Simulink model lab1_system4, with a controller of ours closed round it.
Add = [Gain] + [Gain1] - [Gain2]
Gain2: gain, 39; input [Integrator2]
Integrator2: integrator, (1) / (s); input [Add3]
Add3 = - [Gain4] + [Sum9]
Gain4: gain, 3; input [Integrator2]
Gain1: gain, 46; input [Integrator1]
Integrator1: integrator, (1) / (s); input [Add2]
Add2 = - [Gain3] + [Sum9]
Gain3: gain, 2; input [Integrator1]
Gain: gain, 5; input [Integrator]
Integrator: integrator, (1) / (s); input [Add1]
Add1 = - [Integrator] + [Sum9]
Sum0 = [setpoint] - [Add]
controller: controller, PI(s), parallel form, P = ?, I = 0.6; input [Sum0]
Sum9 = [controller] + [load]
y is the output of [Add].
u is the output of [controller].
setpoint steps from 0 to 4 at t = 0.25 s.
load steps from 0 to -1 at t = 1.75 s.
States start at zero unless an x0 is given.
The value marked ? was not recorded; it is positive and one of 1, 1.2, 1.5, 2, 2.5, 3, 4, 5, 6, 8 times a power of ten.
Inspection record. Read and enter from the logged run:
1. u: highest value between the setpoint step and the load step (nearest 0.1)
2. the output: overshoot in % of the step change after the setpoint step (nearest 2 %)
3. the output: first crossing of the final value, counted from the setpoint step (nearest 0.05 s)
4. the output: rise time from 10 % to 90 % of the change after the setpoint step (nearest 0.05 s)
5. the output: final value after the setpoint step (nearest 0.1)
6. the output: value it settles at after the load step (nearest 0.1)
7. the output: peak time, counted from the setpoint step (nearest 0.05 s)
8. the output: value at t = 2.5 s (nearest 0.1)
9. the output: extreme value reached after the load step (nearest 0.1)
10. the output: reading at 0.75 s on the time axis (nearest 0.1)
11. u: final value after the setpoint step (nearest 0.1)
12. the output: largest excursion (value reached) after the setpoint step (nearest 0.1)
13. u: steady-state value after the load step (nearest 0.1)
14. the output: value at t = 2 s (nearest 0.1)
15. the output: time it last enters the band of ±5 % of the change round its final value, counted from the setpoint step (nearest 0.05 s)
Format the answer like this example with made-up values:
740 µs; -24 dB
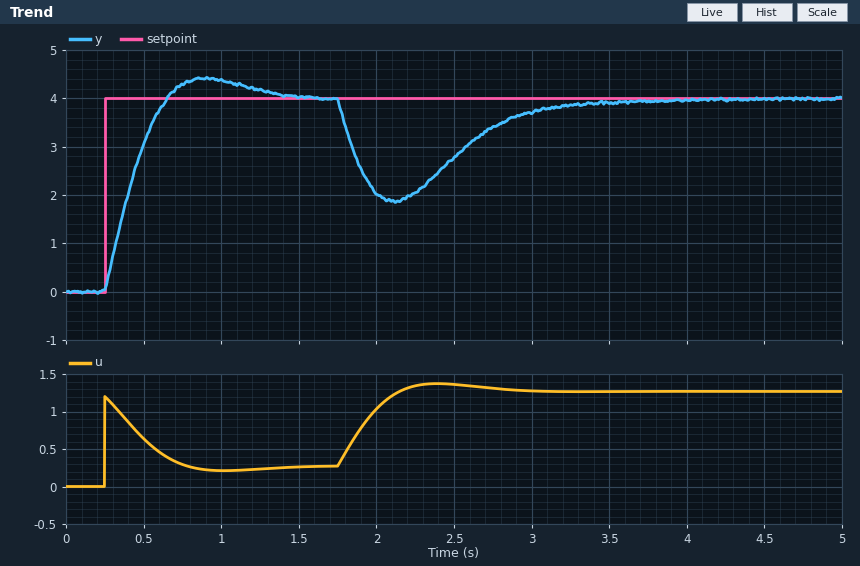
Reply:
1.2; 10 %; 0.40 s; 0.30 s; 4.0; 4.0; 0.65 s; 2.8; 1.9; 4.3; 0.3; 4.4; 1.3; 2.0; 0.95 s
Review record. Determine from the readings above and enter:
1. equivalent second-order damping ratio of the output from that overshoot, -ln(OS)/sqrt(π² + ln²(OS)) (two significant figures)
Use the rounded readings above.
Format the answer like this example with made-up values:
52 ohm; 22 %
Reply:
0.59
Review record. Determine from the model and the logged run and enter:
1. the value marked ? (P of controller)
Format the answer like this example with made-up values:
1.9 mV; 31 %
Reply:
0.3
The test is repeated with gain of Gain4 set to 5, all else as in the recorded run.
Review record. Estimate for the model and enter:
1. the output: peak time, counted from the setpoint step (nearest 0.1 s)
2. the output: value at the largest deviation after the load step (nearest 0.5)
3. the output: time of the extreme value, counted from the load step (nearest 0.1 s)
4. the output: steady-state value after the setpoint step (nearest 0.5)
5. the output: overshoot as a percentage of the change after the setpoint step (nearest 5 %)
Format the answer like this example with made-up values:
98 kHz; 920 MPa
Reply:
0.4 s; 1.5; 0.3 s; 4.0; 15 %
